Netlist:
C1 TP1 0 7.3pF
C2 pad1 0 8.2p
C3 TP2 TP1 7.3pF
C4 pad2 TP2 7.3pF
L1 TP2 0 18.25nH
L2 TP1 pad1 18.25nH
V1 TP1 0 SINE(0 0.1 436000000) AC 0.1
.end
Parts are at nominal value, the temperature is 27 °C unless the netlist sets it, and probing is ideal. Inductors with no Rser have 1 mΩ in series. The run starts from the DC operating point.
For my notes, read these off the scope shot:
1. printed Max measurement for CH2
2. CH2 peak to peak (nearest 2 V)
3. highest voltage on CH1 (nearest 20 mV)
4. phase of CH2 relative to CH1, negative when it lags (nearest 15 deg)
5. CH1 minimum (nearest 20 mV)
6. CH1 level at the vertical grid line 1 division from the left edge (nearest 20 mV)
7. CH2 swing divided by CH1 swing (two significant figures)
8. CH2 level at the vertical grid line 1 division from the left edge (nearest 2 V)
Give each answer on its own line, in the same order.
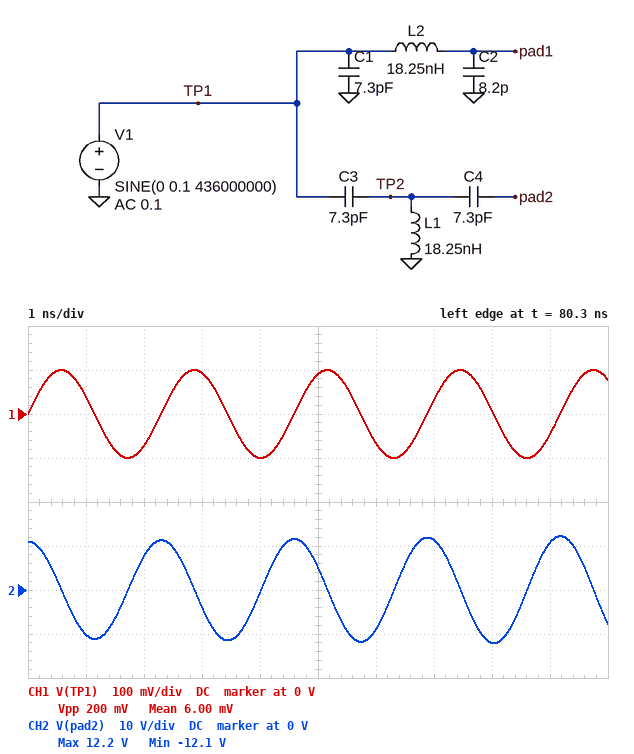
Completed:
12.2 V
24 V
100 mV
90 deg
-100 mV
40 mV
120
-10 V
